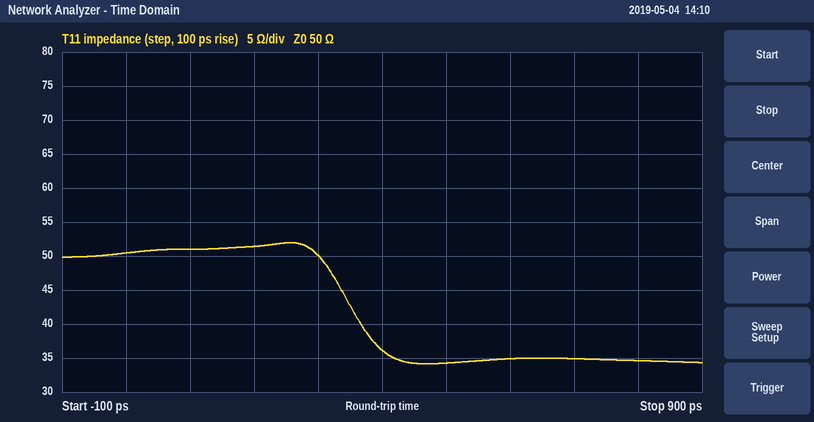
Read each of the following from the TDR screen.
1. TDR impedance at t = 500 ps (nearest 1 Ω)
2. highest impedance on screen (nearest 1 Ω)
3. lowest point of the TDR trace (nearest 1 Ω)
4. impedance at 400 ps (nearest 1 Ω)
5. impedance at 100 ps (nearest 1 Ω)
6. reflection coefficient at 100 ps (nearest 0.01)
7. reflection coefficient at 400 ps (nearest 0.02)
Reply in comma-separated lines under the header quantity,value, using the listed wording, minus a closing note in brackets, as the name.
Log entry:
quantity,value
TDR impedance at t = 500 ps,34 Ω
highest impedance on screen,52 Ω
lowest point of the TDR trace,34 Ω
impedance at 400 ps,36 Ω
impedance at 100 ps,51 Ω
reflection coefficient at 100 ps,+0.01
reflection coefficient at 400 ps,-0.16
